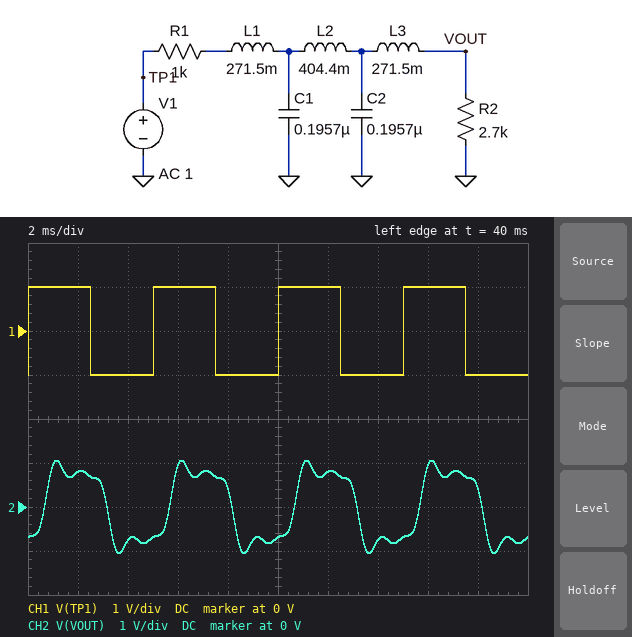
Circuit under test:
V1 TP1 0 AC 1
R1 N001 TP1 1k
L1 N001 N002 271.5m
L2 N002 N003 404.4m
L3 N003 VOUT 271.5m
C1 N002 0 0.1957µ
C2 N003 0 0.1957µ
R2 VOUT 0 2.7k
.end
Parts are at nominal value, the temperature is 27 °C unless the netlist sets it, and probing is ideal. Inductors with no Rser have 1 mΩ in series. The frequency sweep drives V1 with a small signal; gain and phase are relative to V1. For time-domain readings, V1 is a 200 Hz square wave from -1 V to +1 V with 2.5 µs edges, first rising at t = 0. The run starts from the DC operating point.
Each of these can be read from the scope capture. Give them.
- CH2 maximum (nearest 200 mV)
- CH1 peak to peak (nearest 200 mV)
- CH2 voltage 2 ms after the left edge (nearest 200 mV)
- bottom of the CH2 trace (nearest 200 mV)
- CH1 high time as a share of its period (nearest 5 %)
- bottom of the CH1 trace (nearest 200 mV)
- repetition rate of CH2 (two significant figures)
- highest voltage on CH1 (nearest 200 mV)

1.0 V
2.0 V
800 mV
-1.0 V
50 %
-1.0 V
200 Hz
1.0 V
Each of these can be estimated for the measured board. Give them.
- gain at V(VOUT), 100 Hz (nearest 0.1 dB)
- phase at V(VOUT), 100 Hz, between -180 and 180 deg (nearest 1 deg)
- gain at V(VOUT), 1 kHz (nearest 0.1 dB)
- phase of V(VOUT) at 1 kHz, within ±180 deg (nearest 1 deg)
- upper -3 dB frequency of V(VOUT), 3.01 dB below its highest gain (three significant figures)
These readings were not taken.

-2.6 dB
-20 deg
-4.4 dB
79 deg
1.01 kHz
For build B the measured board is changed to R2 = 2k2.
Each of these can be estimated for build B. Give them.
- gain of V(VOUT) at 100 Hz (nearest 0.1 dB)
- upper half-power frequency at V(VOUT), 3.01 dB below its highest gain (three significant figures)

-3.2 dB
1.02 kHz
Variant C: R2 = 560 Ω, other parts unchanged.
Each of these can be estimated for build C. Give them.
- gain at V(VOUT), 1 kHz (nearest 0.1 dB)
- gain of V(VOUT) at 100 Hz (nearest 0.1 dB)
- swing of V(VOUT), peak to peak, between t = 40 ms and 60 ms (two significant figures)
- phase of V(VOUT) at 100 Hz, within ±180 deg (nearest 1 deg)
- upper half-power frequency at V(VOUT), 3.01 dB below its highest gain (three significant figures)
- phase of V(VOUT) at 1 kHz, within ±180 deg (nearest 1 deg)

-8.6 dB
-9.2 dB
900 mV
-26 deg
1.07 kHz
76 deg
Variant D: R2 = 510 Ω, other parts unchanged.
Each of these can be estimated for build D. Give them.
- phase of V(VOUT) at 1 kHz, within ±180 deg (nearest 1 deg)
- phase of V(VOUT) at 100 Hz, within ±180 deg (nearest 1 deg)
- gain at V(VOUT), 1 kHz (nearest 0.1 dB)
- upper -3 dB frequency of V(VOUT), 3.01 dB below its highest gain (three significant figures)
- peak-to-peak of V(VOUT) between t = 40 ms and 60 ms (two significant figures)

76 deg
-27 deg
-9.0 dB
1.07 kHz
840 mV
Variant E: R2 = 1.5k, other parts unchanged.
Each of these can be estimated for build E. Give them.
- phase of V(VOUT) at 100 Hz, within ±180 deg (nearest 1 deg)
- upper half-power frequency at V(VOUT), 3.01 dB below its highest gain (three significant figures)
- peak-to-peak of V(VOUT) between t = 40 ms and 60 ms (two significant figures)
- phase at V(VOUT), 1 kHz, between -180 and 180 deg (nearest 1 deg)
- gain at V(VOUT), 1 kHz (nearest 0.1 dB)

-22 deg
1.04 kHz
1.6 V
78 deg
-5.5 dB
